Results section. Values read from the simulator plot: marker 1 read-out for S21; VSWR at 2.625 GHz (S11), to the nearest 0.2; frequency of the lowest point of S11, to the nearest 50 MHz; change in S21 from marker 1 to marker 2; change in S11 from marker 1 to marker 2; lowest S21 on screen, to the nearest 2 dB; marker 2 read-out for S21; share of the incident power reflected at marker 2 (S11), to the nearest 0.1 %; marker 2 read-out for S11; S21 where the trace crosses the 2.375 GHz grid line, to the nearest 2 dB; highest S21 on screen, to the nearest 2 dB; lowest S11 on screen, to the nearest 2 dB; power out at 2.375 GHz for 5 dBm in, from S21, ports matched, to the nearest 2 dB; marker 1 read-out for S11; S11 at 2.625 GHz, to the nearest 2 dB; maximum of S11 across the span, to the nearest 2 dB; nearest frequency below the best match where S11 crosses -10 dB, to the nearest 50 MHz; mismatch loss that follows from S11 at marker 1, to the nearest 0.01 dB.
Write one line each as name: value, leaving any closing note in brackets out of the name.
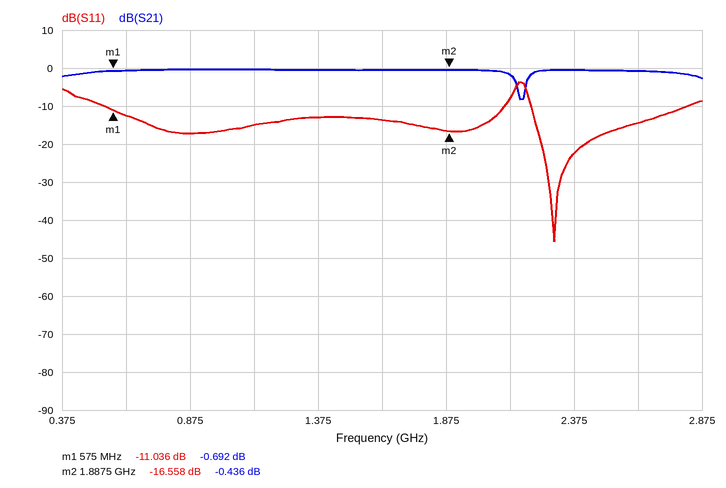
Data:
marker 1 read-out for S21: -0.692 dB
VSWR at 2.625 GHz (S11), to the nearest 0.2: 1.4
frequency of the lowest point of S11, to the nearest 50 MHz: 2.30 GHz
change in S21 from marker 1 to marker 2: 0.256 dB
change in S11 from marker 1 to marker 2: -5.522 dB
lowest S21 on screen, to the nearest 2 dB: -8 dB
marker 2 read-out for S21: -0.436 dB
share of the incident power reflected at marker 2 (S11), to the nearest 0.1 %: 2.2 %
marker 2 read-out for S11: -16.558 dB
S21 where the trace crosses the 2.375 GHz grid line, to the nearest 2 dB: 0 dB
highest S21 on screen, to the nearest 2 dB: 0 dB
lowest S11 on screen, to the nearest 2 dB: -46 dB
power out at 2.375 GHz for 5 dBm in, from S21, ports matched, to the nearest 2 dB: 4 dBm
marker 1 read-out for S11: -11.036 dB
S11 at 2.625 GHz, to the nearest 2 dB: -14 dB
maximum of S11 across the span, to the nearest 2 dB: -4 dB
nearest frequency below the best match where S11 crosses -10 dB, to the nearest 50 MHz: 2.20 GHz
mismatch loss that follows from S11 at marker 1, to the nearest 0.01 dB: 0.36 dB
